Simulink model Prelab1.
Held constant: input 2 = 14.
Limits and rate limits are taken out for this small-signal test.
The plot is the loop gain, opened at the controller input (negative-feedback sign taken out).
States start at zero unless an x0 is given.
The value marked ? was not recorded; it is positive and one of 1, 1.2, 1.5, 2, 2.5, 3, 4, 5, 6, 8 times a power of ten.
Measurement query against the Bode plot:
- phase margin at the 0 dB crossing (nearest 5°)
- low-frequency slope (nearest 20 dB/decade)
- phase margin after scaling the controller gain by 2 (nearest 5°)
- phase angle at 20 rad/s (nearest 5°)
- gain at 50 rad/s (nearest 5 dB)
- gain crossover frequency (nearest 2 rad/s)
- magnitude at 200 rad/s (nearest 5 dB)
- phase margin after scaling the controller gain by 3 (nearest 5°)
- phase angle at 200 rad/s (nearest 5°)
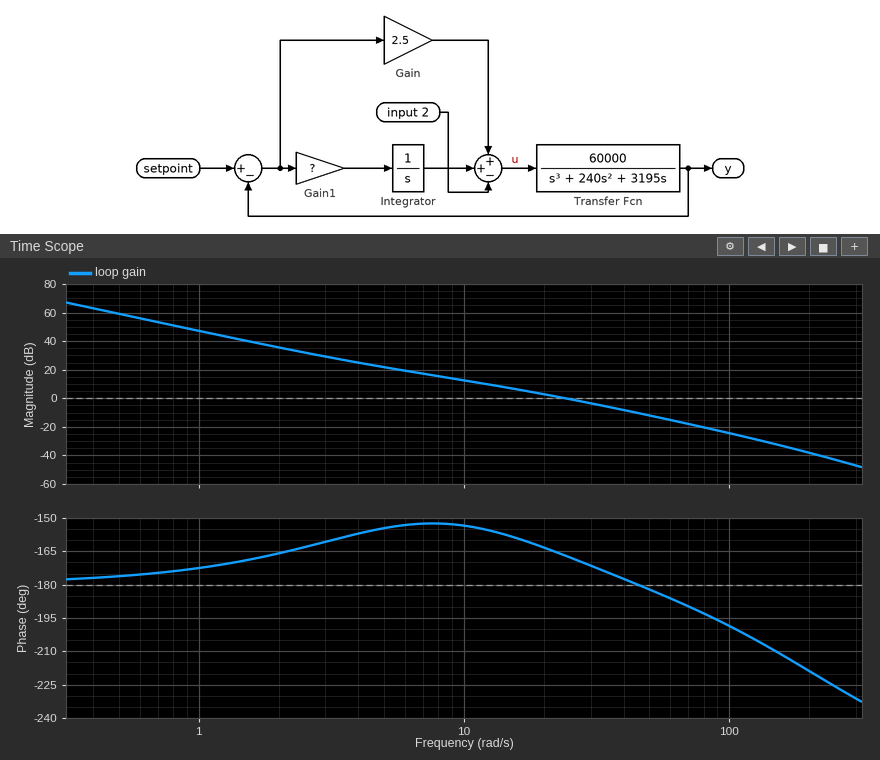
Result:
15°
-40 dB/decade
5°
-165°
-10 dB
24 rad/s
-40 dB
0°
-220°
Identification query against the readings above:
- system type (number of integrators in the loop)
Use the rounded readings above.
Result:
2
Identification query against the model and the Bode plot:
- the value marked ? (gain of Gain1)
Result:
12
